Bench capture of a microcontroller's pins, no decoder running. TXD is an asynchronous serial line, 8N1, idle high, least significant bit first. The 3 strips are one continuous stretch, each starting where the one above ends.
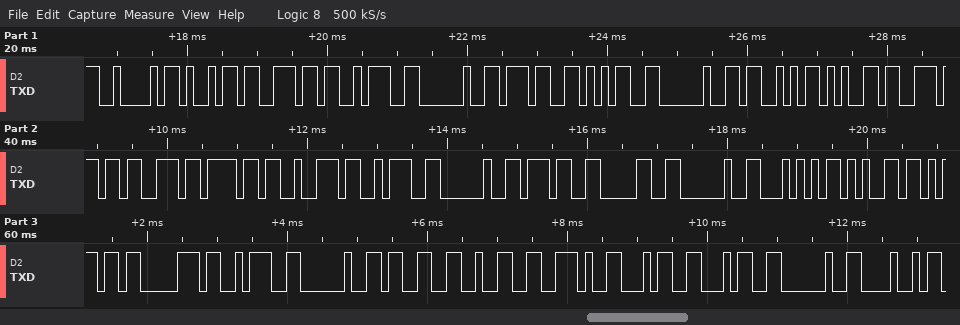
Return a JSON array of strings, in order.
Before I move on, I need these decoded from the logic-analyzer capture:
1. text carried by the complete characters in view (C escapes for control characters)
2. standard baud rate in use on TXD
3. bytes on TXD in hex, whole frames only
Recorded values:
["\"Bin: 75 Sensor: 70 Temp: 32.44 H\"", "9600 baud", "42 69 6E 3A 20 37 35 20 53 65 6E 73 6F 72 3A 20 37 30 20 54 65 6D 70 3A 20 33 32 2E 34 34 20 48"]
